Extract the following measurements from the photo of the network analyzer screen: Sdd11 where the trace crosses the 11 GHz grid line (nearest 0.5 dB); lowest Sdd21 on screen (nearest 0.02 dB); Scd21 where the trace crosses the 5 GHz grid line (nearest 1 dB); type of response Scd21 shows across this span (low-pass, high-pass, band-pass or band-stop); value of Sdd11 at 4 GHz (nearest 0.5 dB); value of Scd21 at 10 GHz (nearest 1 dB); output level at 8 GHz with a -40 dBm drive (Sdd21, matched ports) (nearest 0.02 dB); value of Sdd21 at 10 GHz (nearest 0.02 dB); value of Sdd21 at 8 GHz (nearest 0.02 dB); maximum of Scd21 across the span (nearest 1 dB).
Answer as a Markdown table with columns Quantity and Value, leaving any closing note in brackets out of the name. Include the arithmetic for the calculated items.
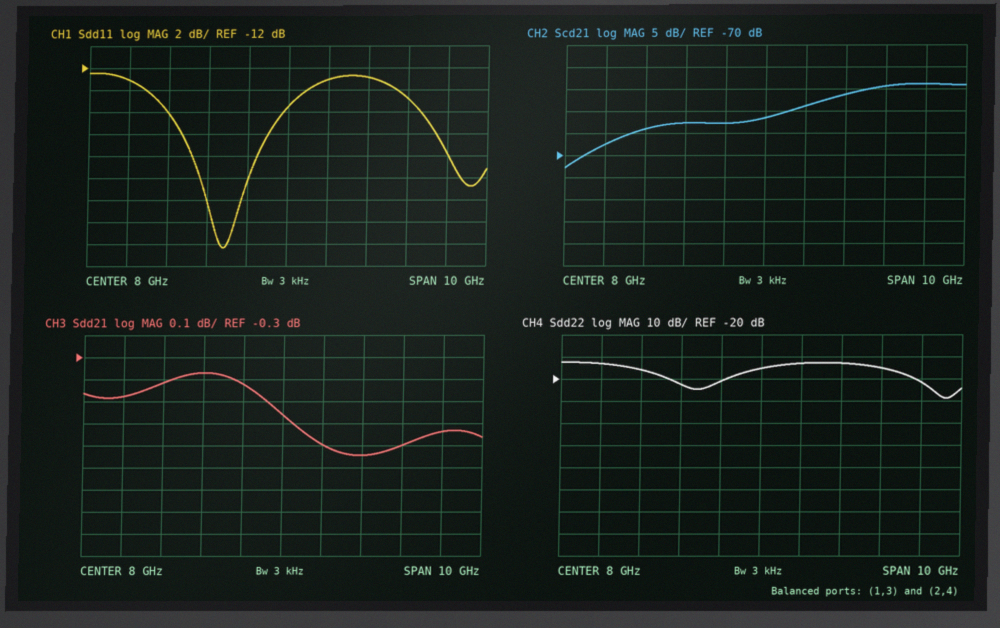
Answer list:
| Quantity | Value |
|---|---|
| Sdd11 where the trace crosses the 11 GHz grid line | -15.0 dB |
| lowest Sdd21 on screen | -0.74 dB |
| Scd21 where the trace crosses the 5 GHz grid line | -64 dB |
| type of response Scd21 shows across this span | high-pass |
| value of Sdd11 at 4 GHz | -13.0 dB |
| value of Scd21 at 10 GHz | -56 dB |
| output level at 8 GHz with a -40 dBm drive (Sdd21, matched ports) | -40 dBm + (-0.56 dB) = -40.56 dBm |
| value of Sdd21 at 10 GHz | -0.74 dB |
| value of Sdd21 at 8 GHz | -0.56 dB |
| maximum of Scd21 across the span | -54 dB |
